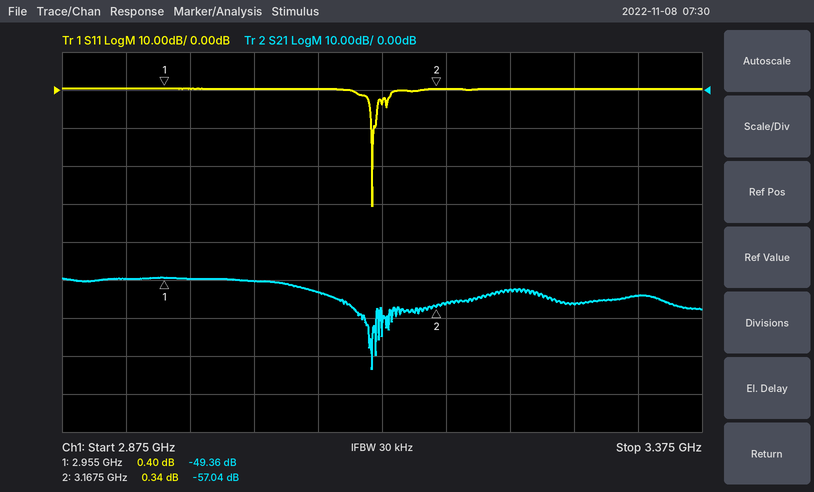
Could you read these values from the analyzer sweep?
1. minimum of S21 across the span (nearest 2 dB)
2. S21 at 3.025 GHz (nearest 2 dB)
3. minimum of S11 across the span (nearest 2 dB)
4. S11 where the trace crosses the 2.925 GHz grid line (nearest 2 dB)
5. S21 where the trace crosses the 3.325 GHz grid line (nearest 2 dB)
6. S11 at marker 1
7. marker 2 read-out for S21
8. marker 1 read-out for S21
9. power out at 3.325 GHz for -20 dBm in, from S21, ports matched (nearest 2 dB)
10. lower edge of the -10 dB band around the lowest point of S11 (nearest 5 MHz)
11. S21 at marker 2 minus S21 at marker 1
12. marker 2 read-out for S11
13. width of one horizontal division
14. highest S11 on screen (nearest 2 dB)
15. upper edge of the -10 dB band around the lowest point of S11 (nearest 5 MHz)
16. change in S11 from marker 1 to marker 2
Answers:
-74 dB
-50 dB
-30 dB
0 dB
-54 dB
0.40 dB
-57.04 dB
-49.36 dB
-74 dBm
3.115 GHz
-7.68 dB
0.34 dB
50 MHz
0 dB
3.120 GHz
-0.06 dB
